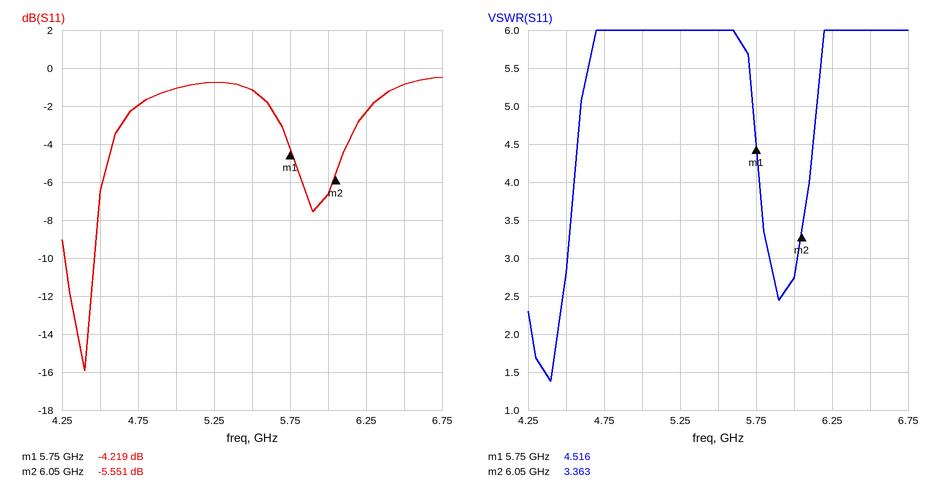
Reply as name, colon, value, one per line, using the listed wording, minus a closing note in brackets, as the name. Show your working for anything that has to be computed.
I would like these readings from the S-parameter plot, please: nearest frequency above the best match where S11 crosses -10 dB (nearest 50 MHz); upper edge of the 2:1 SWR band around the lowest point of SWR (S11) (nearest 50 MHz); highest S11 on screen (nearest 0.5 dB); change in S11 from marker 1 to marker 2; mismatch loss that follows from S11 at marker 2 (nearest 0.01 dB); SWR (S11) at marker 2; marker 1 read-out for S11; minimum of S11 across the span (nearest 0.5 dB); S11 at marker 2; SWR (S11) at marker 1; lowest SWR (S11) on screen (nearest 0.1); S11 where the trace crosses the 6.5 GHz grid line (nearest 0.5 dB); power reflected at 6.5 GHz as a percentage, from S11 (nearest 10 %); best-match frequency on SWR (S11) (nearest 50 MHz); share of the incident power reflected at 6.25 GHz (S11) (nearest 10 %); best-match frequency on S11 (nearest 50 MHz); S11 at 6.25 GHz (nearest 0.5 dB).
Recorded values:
nearest frequency above the best match where S11 crosses -10 dB: 4.45 GHz
upper edge of the 2:1 SWR band around the lowest point of SWR (S11): 4.45 GHz
highest S11 on screen: -0.5 dB
change in S11 from marker 1 to marker 2: -5.551 − (-4.219) = -1.332 dB
mismatch loss that follows from S11 at marker 2: −10 log10(1 − 10^(-5.551/10)) ≈ 1.42 dB
SWR (S11) at marker 2: 3.363
marker 1 read-out for S11: -4.219 dB
minimum of S11 across the span: -16.0 dB
S11 at marker 2: -5.551 dB
SWR (S11) at marker 1: 4.516
lowest SWR (S11) on screen: 1.4
S11 where the trace crosses the 6.5 GHz grid line: -1.0 dB
power reflected at 6.5 GHz as a percentage, from S11: 10^(-1/10) ≈ 79.4 %, so 80 % to the nearest 10 %
best-match frequency on SWR (S11): 4.40 GHz
share of the incident power reflected at 6.25 GHz (S11): 10^(-2.5/10) ≈ 56.2 %, so 60 % to the nearest 10 %
best-match frequency on S11: 4.40 GHz
S11 at 6.25 GHz: -2.5 dB
